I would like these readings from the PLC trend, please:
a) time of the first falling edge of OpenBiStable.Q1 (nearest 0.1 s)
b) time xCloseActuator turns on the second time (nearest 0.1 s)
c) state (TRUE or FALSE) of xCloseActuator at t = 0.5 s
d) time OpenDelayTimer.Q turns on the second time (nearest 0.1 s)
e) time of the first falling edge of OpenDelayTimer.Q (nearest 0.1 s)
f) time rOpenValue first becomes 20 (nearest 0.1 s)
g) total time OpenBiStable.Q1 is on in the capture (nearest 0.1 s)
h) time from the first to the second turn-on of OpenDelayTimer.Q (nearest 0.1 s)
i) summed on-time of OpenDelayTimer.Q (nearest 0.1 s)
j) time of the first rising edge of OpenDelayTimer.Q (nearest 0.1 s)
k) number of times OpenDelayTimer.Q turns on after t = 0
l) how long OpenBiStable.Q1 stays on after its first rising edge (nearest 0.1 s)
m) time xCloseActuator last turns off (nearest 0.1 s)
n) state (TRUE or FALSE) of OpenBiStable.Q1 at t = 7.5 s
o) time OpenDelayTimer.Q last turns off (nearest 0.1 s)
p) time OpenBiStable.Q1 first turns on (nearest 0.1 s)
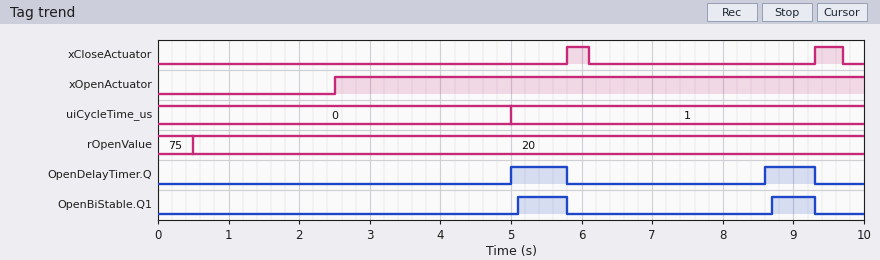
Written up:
5.8 s
9.3 s
FALSE
8.6 s
5.8 s
0.5 s
1.3 s
3.6 s
1.5 s
5.0 s
2
0.7 s
9.7 s
FALSE
9.3 s
5.1 s
